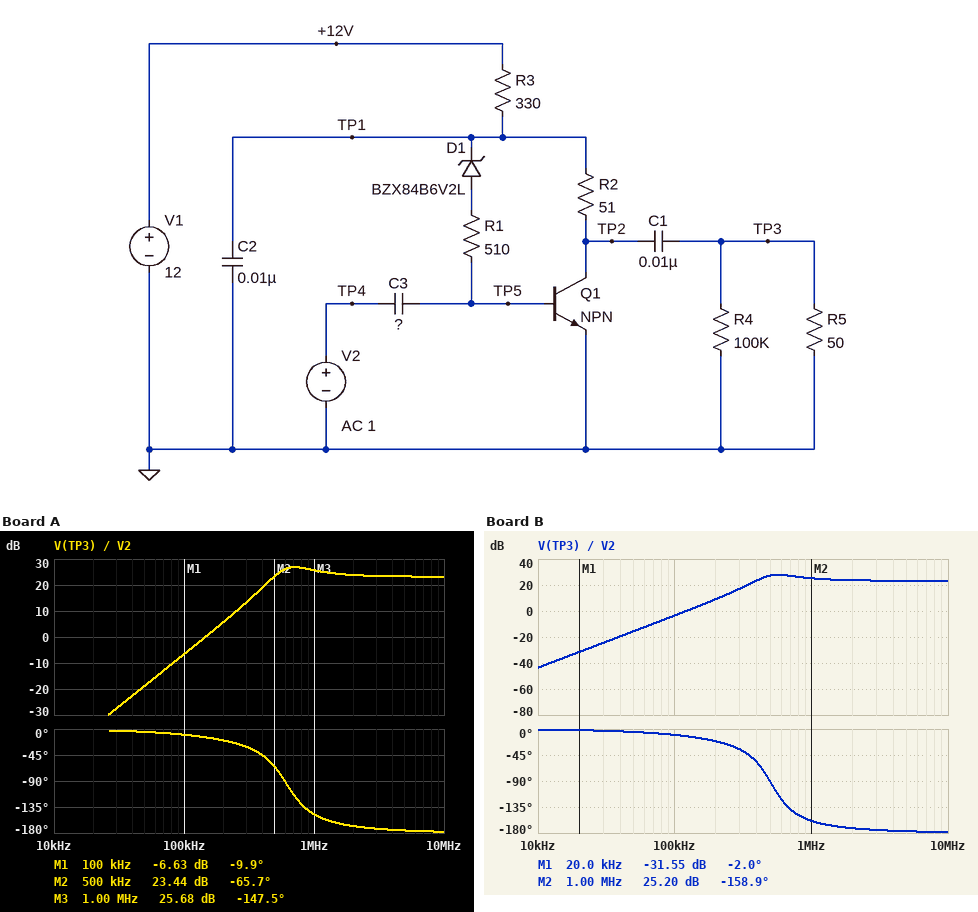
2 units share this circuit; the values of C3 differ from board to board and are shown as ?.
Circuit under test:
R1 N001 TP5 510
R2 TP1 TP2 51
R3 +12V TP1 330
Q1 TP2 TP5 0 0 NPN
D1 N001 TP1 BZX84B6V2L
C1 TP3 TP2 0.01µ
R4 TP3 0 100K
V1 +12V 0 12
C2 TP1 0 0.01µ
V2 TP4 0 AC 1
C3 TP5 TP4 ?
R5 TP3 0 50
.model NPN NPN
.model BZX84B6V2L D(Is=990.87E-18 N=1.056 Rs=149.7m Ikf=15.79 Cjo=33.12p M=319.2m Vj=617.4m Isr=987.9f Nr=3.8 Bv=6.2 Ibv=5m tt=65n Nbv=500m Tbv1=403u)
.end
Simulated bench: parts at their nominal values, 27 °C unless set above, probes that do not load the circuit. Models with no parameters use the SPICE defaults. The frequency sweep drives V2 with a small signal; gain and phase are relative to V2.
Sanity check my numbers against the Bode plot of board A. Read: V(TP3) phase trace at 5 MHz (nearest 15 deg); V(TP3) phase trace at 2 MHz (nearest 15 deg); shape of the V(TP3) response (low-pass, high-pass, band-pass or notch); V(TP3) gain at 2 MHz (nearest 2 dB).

-180 deg
-165 deg
high-pass
24 dB
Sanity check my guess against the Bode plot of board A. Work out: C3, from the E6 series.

3.3 nF
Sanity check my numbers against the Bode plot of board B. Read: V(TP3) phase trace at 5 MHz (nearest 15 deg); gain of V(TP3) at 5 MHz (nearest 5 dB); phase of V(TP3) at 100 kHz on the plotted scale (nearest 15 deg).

-180 deg
25 dB
-15 deg
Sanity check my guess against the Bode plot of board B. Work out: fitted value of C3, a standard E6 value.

4.7 nF
